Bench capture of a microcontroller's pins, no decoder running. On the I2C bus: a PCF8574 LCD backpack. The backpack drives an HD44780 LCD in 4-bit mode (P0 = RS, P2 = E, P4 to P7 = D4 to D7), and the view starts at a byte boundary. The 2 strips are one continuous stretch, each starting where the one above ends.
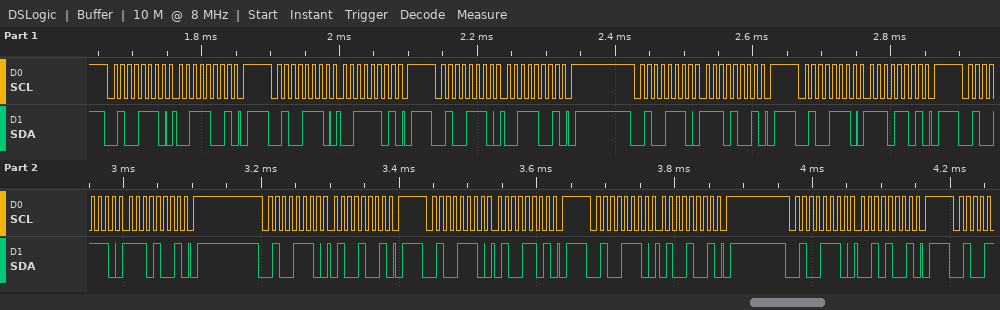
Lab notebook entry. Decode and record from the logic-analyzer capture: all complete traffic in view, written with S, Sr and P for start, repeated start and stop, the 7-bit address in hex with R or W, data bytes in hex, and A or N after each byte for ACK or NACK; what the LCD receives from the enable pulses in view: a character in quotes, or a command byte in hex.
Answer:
S 27W A 39 A P S 27W A 3D A P S 27W A 39 A P S 27W A E9 A P S 27W A ED A P S 27W A E9 A P S 27W A 49 A P S 27W A 4D A P S 27W A 49 A P S 27W A 29 A P
'>'
